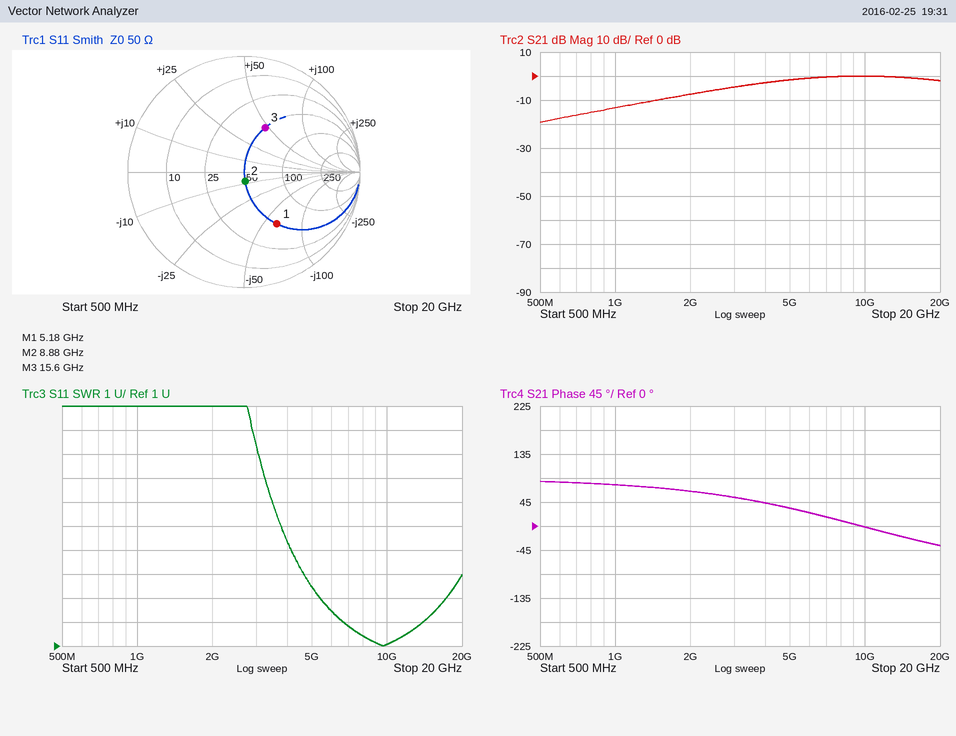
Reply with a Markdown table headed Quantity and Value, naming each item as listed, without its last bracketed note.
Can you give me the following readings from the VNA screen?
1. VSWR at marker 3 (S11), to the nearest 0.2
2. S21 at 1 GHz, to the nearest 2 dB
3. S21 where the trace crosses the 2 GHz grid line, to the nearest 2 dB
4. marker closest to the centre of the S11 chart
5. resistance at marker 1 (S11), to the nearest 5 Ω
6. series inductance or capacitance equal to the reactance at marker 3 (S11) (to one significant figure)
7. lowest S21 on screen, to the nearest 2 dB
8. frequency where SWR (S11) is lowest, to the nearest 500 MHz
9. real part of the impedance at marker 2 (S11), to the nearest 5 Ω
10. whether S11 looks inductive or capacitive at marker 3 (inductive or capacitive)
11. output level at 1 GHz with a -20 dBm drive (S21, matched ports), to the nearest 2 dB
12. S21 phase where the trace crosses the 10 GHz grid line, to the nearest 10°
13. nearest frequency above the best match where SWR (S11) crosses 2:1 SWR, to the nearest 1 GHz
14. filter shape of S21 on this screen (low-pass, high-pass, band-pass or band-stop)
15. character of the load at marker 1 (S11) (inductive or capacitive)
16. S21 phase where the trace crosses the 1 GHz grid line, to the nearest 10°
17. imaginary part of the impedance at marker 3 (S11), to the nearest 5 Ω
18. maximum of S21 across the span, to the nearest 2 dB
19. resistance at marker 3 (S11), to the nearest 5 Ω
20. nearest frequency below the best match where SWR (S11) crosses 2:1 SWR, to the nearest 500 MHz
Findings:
| Quantity | Value |
|---|---|
| VSWR at marker 3 (S11), to the nearest 0.2 | 2.4 |
| S21 at 1 GHz, to the nearest 2 dB | -14 dB |
| S21 where the trace crosses the 2 GHz grid line, to the nearest 2 dB | -8 dB |
| marker closest to the centre of the S11 chart | marker 2 |
| resistance at marker 1 (S11), to the nearest 5 Ω | 50 Ω |
| series inductance or capacitance equal to the reactance at marker 3 (S11) | 500 pH |
| lowest S21 on screen, to the nearest 2 dB | -20 dB |
| frequency where SWR (S11) is lowest, to the nearest 500 MHz | 9.5 GHz |
| real part of the impedance at marker 2 (S11), to the nearest 5 Ω | 50 Ω |
| whether S11 looks inductive or capacitive at marker 3 | inductive |
| output level at 1 GHz with a -20 dBm drive (S21, matched ports), to the nearest 2 dB | -34 dBm |
| S21 phase where the trace crosses the 10 GHz grid line, to the nearest 10° | 0° |
| nearest frequency above the best match where SWR (S11) crosses 2:1 SWR, to the nearest 1 GHz | 14 GHz |
| filter shape of S21 on this screen | high-pass |
| character of the load at marker 1 (S11) | capacitive |
| S21 phase where the trace crosses the 1 GHz grid line, to the nearest 10° | 80° |
| imaginary part of the impedance at marker 3 (S11), to the nearest 5 Ω | +45 Ω |
| maximum of S21 across the span, to the nearest 2 dB | 0 dB |
| resistance at marker 3 (S11), to the nearest 5 Ω | 50 Ω |
| nearest frequency below the best match where SWR (S11) crosses 2:1 SWR, to the nearest 500 MHz | 6.5 GHz |
